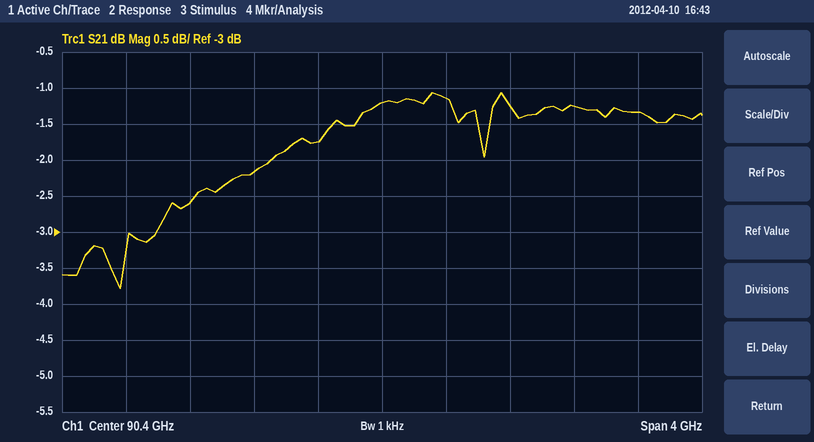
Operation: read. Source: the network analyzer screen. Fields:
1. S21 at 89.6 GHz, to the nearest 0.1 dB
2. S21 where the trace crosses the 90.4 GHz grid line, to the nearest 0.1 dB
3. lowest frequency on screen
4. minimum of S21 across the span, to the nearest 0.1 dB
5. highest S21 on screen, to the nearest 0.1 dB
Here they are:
-2.2 dB
-1.2 dB
88.4 GHz
-3.8 dB
-1.1 dB
